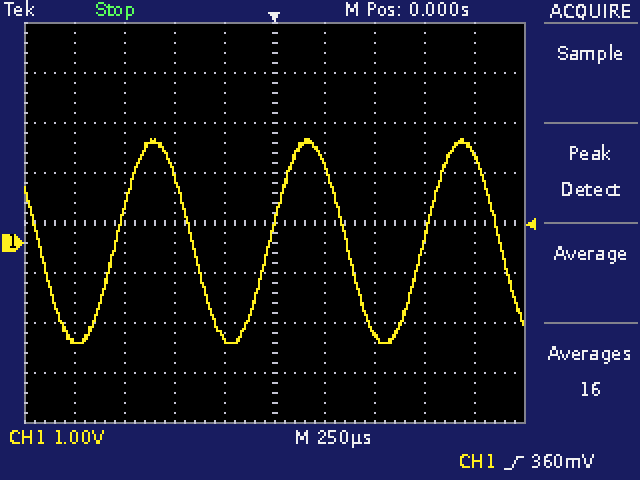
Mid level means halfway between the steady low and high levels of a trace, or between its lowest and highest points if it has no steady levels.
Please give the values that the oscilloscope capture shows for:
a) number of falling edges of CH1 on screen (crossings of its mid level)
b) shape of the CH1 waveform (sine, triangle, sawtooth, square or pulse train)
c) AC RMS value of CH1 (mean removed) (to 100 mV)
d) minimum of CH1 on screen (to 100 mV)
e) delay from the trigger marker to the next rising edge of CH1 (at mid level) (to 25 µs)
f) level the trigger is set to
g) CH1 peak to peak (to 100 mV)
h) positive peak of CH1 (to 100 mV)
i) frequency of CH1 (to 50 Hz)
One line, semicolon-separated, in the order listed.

4; sine; 1.4 V; -2.0 V; 750 µs; 360 mV; 4.1 V; 2.1 V; 1.30 kHz
